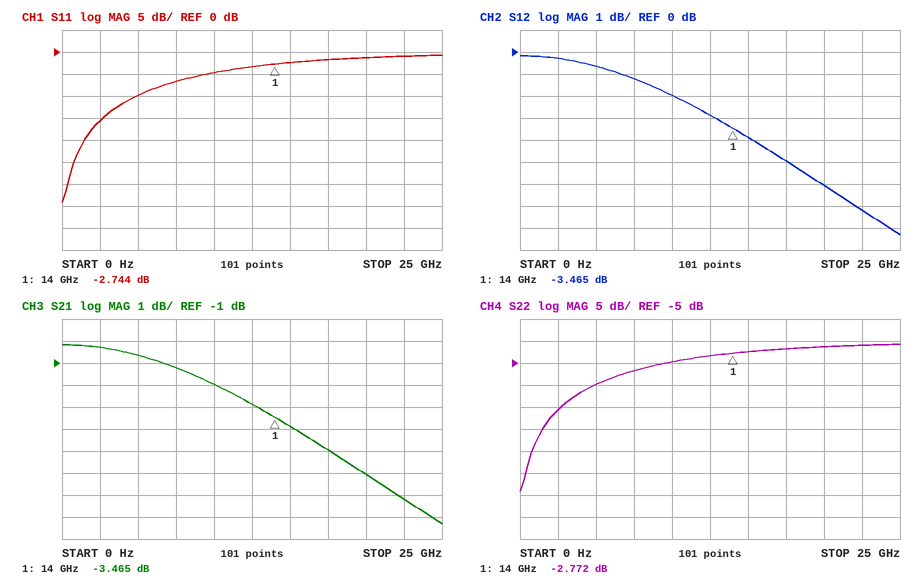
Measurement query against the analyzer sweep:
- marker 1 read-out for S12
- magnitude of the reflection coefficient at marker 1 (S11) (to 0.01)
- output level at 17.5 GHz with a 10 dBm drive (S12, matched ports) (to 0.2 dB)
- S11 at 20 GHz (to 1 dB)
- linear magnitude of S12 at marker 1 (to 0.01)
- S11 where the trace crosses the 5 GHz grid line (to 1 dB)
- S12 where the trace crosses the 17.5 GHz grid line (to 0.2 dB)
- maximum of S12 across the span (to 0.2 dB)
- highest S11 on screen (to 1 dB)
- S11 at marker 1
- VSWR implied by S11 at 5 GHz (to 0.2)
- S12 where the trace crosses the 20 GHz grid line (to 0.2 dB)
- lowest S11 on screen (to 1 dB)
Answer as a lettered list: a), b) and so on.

a) -3.465 dB
b) 0.73
c) 5.0 dBm
d) -1 dB
e) 0.67
f) -10 dB
g) -5.0 dB
h) -0.2 dB
i) -1 dB
j) -2.744 dB
k) 2.0
l) -6.0 dB
m) -34 dB
